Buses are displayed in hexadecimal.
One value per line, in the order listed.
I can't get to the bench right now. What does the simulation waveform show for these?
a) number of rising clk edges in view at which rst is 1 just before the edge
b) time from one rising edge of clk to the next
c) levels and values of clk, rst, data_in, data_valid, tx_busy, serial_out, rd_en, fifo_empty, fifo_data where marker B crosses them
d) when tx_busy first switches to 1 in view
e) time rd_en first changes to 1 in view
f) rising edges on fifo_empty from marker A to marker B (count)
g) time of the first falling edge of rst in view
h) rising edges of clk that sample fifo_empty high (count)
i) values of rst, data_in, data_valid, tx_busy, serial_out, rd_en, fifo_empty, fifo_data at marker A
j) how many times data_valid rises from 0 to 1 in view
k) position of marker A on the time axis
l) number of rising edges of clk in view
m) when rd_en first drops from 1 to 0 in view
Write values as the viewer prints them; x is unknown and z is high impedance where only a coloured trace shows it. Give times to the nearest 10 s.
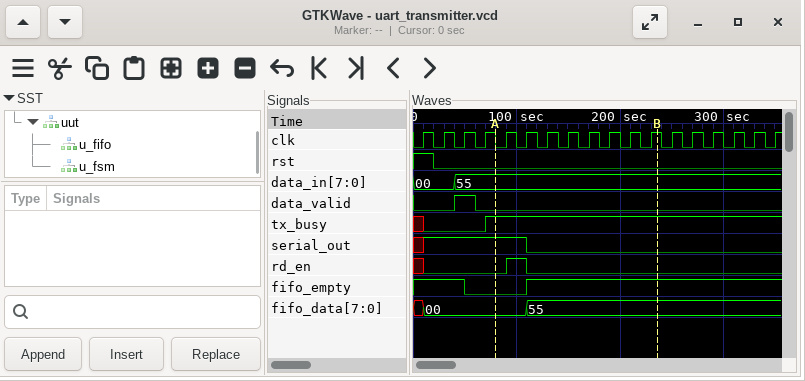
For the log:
1
20 s
clk=1, rst=0, data_in=55, data_valid=0, tx_busy=1, serial_out=0, rd_en=0, fifo_empty=1, fifo_data=55
70 s
90 s
1
20 s
15
rst=0, data_in=55, data_valid=0, tx_busy=1, serial_out=1, rd_en=0, fifo_empty=0, fifo_data=00
1
80 s
18
110 s
